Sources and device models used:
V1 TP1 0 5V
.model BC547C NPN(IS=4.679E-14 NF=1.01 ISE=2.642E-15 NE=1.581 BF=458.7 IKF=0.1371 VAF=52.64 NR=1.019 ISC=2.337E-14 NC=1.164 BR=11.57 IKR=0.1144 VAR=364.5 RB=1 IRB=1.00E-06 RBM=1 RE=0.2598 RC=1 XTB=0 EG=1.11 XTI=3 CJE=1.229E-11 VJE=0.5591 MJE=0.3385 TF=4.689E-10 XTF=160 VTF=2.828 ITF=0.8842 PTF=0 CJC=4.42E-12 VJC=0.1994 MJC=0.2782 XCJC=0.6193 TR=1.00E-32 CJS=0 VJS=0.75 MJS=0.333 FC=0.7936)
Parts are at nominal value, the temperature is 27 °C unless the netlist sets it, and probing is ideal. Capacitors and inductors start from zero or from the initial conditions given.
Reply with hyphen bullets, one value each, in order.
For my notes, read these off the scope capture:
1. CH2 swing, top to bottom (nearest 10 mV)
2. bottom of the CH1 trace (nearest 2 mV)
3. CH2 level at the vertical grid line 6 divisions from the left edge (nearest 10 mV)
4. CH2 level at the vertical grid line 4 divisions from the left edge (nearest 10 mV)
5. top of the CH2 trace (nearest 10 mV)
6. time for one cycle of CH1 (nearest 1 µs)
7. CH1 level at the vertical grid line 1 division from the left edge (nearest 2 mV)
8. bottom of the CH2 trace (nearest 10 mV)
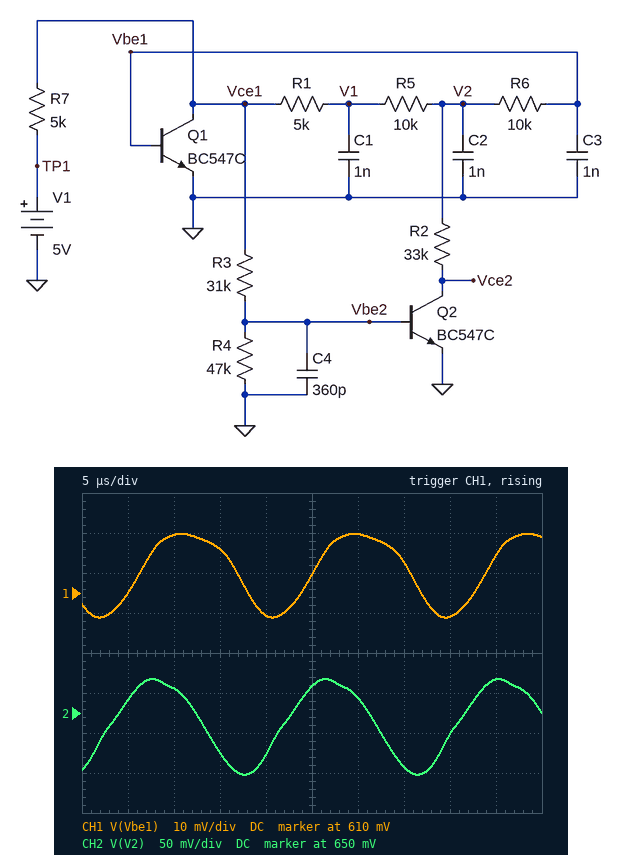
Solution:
- 120 mV
- 604 mV
- 670 mV
- 600 mV
- 690 mV
- 19 µs
- 610 mV
- 570 mV
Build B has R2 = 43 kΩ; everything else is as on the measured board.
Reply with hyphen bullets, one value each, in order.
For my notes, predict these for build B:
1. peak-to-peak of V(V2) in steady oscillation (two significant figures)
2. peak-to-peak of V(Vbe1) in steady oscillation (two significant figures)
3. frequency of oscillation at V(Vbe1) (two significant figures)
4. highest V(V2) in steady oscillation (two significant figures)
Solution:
- 130 mV
- 22 mV
- 54 kHz
- 700 mV
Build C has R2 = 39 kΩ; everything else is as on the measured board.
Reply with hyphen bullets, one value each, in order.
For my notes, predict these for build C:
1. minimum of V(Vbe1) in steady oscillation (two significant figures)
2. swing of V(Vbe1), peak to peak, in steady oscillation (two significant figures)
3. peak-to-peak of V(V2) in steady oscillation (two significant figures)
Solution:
- 600 mV
- 22 mV
- 130 mV
